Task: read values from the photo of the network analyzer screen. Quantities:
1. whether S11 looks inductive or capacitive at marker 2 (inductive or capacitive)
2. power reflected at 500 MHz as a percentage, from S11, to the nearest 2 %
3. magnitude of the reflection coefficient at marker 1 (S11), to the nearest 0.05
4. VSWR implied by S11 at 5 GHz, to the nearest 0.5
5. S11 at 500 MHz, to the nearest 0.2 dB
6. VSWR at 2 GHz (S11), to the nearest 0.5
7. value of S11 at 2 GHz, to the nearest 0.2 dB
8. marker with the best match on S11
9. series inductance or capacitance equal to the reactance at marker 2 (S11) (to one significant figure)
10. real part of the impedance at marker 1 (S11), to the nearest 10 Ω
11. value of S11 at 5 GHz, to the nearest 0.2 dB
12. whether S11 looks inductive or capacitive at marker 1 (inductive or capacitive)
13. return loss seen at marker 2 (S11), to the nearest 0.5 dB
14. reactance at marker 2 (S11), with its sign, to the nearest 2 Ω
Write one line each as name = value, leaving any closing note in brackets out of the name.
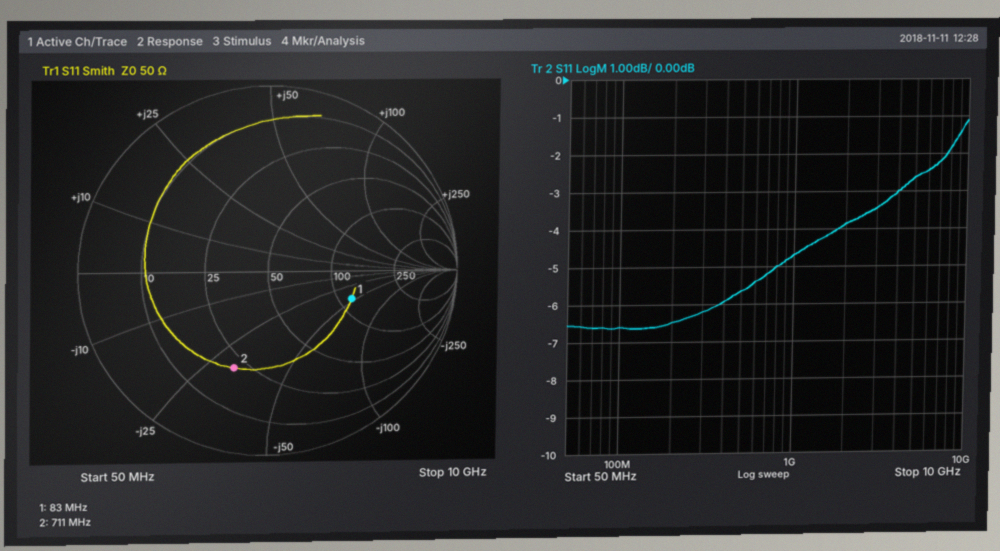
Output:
whether S11 looks inductive or capacitive at marker 2 = capacitive
power reflected at 500 MHz as a percentage, from S11, to the nearest 2 % = 28 %
magnitude of the reflection coefficient at marker 1 (S11), to the nearest 0.05 = 0.45
VSWR implied by S11 at 5 GHz, to the nearest 0.5 = 6.5
S11 at 500 MHz, to the nearest 0.2 dB = -5.6 dB
VSWR at 2 GHz (S11), to the nearest 0.5 = 4.5
value of S11 at 2 GHz, to the nearest 0.2 dB = -3.8 dB
marker with the best match on S11 = marker 1
series inductance or capacitance equal to the reactance at marker 2 (S11) = 7 pF
real part of the impedance at marker 1 (S11), to the nearest 10 Ω = 120 Ω
value of S11 at 5 GHz, to the nearest 0.2 dB = -2.6 dB
whether S11 looks inductive or capacitive at marker 1 = capacitive
return loss seen at marker 2 (S11), to the nearest 0.5 dB = 5.0 dB
reactance at marker 2 (S11), with its sign, to the nearest 2 Ω = -32 Ω
